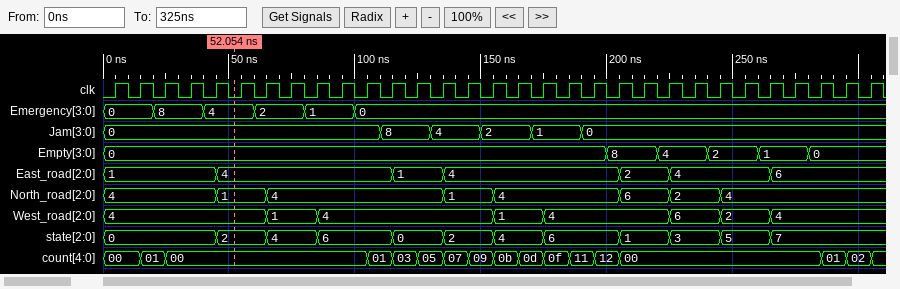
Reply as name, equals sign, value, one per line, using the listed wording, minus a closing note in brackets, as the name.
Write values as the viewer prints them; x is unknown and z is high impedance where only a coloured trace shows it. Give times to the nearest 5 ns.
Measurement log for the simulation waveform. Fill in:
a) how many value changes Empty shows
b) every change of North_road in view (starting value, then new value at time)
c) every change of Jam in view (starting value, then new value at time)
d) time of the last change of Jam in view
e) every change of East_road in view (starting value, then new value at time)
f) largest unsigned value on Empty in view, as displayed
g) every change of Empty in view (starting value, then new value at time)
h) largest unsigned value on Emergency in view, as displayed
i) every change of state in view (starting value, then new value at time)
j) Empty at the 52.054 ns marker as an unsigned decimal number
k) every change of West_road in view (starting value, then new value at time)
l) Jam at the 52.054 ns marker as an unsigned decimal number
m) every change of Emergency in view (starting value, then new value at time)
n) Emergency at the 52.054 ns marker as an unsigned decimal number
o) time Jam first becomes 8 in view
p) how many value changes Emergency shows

how many value changes Empty shows = 5
every change of North_road in view = 4, 1 at 45 ns, 4 at 65 ns, 1 at 135 ns, 4 at 155 ns, 6 at 205 ns, 2 at 225 ns, 4 at 245 ns
every change of Jam in view = 0, 8 at 110 ns, 4 at 130 ns, 2 at 150 ns, 1 at 170 ns, 0 at 190 ns
time of the last change of Jam in view = 190 ns
every change of East_road in view = 1, 4 at 45 ns, 1 at 115 ns, 4 at 135 ns, 2 at 205 ns, 4 at 225 ns, 6 at 265 ns
largest unsigned value on Empty in view, as displayed = 8
every change of Empty in view = 0, 8 at 200 ns, 4 at 220 ns, 2 at 240 ns, 1 at 260 ns, 0 at 280 ns
largest unsigned value on Emergency in view, as displayed = 8
every change of state in view = 0, 2 at 45 ns, 4 at 65 ns, 6 at 85 ns, 0 at 115 ns, 2 at 135 ns, 4 at 155 ns, 6 at 175 ns, 1 at 205 ns, 3 at 225 ns, 5 at 245 ns, 7 at 265 ns
Empty at the 52.054 ns marker as an unsigned decimal number = 0
every change of West_road in view = 4, 1 at 65 ns, 4 at 85 ns, 1 at 155 ns, 4 at 175 ns, 6 at 225 ns, 2 at 245 ns, 4 at 265 ns
Jam at the 52.054 ns marker as an unsigned decimal number = 0
every change of Emergency in view = 0, 8 at 20 ns, 4 at 40 ns, 2 at 60 ns, 1 at 80 ns, 0 at 100 ns
Emergency at the 52.054 ns marker as an unsigned decimal number = 4
time Jam first becomes 8 in view = 110 ns
how many value changes Emergency shows = 5
